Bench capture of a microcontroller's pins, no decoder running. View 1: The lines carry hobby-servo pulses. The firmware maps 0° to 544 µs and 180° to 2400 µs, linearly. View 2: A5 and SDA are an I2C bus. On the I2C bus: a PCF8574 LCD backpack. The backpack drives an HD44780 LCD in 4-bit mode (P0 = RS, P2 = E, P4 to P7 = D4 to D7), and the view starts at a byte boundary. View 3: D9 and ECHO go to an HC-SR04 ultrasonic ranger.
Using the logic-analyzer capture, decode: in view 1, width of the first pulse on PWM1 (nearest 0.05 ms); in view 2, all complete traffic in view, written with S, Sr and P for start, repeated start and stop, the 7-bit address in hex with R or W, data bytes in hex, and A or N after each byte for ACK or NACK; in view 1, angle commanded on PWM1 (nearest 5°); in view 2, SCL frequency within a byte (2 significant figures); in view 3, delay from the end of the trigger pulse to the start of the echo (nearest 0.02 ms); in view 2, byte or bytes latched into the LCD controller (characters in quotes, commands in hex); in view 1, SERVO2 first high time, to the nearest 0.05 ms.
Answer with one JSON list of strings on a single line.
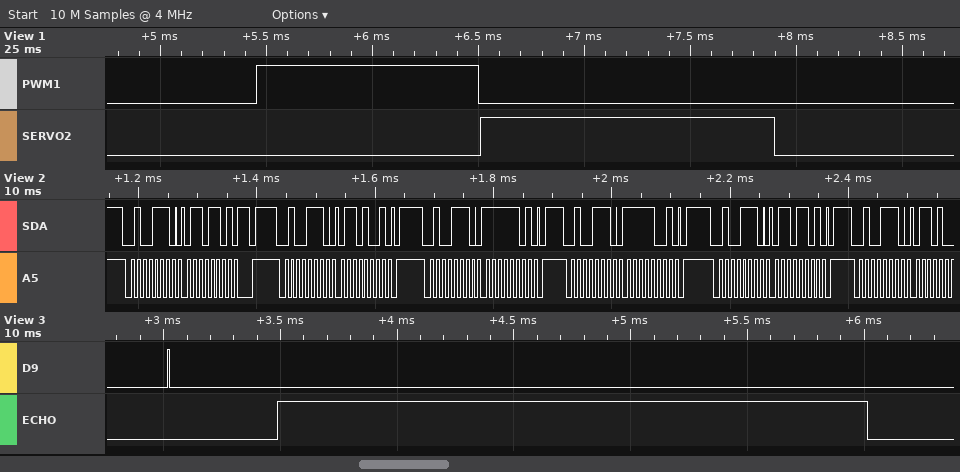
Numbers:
["1.05 ms", "S 27W A 6D A P S 27W A 69 A P S 27W A FD A P S 27W A F9 A P S 27W A 6D A P S 27W A", "50°", "100 kHz", "0.46 ms", "'o'", "1.40 ms"]
